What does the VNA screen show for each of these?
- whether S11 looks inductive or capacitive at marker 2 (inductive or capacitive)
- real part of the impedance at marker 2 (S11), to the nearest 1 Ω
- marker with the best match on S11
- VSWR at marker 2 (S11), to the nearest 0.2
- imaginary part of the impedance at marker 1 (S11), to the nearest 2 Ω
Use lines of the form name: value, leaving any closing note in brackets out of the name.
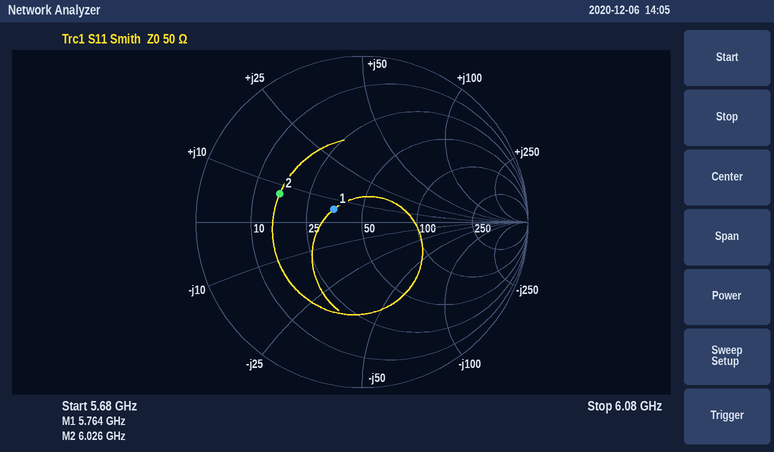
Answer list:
whether S11 looks inductive or capacitive at marker 2: inductive
real part of the impedance at marker 2 (S11), to the nearest 1 Ω: 16 Ω
marker with the best match on S11: marker 1
VSWR at marker 2 (S11), to the nearest 0.2: 3.2
imaginary part of the impedance at marker 1 (S11), to the nearest 2 Ω: +6 Ω
